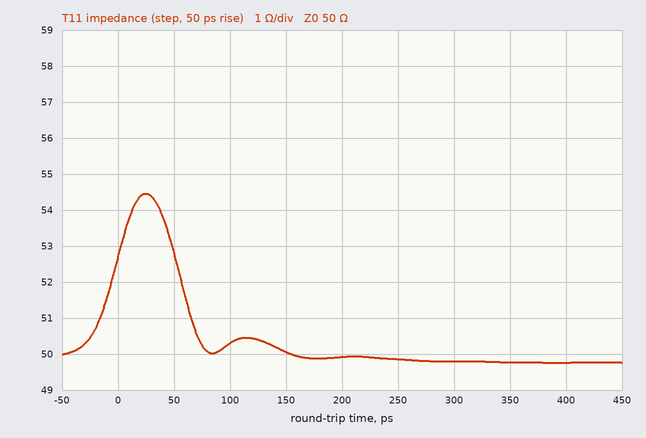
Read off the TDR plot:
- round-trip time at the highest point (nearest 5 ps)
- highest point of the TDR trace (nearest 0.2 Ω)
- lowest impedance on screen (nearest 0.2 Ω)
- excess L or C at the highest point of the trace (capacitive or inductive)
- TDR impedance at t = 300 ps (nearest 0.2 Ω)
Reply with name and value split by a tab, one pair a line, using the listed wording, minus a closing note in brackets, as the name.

round-trip time at the highest point	25 ps
highest point of the TDR trace	54.4 Ω
lowest impedance on screen	49.8 Ω
excess L or C at the highest point of the trace	inductive
TDR impedance at t = 300 ps	49.8 Ω
